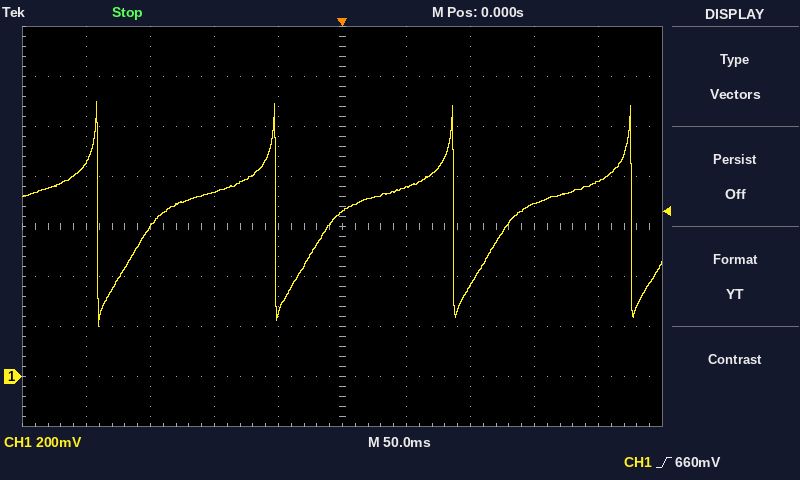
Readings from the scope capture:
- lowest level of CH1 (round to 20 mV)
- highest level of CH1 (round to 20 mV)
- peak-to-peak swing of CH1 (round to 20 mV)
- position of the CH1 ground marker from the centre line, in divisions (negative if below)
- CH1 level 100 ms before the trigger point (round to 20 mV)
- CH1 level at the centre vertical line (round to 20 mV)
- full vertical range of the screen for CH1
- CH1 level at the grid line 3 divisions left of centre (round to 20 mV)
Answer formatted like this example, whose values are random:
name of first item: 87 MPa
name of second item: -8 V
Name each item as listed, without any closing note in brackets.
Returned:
lowest level of CH1: 200 mV
highest level of CH1: 1.10 V
peak-to-peak swing of CH1: 900 mV
position of the CH1 ground marker from the centre line, in divisions: -3.0 div
CH1 level 100 ms before the trigger point: 740 mV
CH1 level at the centre vertical line: 660 mV
full vertical range of the screen for CH1: 1.6 V
CH1 level at the grid line 3 divisions left of centre: 600 mV
